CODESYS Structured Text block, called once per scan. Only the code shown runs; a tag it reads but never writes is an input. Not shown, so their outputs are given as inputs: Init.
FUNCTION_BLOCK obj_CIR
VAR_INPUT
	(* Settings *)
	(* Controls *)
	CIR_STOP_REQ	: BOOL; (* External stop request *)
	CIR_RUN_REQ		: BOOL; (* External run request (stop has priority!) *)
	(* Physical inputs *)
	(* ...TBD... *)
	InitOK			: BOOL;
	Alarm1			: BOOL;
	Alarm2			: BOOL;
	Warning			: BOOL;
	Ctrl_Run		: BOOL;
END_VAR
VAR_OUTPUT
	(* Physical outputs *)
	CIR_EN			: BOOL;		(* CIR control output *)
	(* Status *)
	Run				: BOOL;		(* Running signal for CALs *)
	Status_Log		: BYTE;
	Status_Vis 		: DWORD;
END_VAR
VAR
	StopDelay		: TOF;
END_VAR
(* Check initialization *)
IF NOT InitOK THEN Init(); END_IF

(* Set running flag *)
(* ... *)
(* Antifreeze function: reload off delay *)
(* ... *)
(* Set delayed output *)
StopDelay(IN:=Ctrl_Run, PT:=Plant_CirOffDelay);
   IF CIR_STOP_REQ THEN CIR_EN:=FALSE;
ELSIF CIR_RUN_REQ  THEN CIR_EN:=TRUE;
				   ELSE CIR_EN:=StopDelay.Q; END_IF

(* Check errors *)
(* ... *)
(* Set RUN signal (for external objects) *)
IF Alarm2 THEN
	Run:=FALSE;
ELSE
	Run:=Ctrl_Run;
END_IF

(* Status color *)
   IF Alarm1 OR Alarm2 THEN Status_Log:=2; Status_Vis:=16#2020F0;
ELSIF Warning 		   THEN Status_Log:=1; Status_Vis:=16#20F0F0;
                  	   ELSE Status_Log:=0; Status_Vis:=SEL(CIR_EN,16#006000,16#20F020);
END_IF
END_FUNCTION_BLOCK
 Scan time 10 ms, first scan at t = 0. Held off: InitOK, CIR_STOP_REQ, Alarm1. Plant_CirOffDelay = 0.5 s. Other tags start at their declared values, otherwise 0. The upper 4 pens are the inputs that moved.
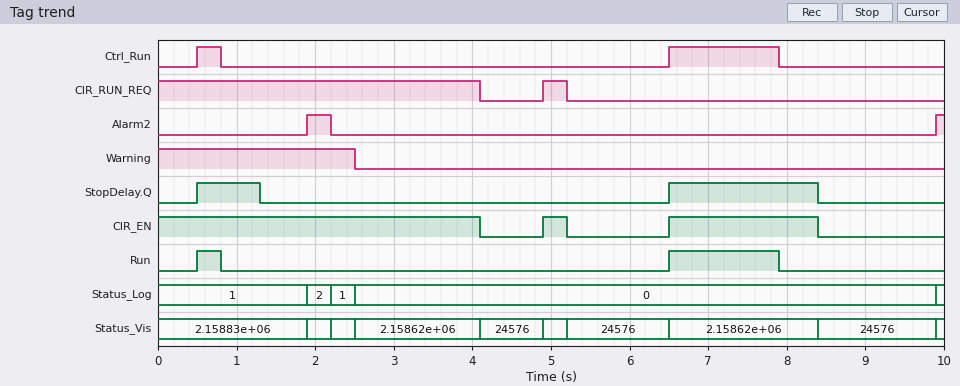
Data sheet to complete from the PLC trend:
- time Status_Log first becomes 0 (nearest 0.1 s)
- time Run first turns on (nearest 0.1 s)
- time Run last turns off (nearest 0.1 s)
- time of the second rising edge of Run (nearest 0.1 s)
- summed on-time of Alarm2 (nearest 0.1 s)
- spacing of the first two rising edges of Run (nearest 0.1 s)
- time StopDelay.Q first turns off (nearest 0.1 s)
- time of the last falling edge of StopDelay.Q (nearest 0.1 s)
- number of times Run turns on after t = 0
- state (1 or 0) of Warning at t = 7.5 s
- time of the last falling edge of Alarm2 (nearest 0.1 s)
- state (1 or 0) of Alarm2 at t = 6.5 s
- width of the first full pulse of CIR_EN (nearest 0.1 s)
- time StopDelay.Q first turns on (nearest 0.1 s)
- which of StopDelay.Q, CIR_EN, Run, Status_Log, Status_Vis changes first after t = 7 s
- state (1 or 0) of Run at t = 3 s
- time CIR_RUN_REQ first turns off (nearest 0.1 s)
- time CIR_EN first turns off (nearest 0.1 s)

2.5 s
0.5 s
7.9 s
6.5 s
0.4 s
6.0 s
1.3 s
8.4 s
2
0
2.2 s
0
0.3 s
0.5 s
Run
0
4.1 s
4.1 s
